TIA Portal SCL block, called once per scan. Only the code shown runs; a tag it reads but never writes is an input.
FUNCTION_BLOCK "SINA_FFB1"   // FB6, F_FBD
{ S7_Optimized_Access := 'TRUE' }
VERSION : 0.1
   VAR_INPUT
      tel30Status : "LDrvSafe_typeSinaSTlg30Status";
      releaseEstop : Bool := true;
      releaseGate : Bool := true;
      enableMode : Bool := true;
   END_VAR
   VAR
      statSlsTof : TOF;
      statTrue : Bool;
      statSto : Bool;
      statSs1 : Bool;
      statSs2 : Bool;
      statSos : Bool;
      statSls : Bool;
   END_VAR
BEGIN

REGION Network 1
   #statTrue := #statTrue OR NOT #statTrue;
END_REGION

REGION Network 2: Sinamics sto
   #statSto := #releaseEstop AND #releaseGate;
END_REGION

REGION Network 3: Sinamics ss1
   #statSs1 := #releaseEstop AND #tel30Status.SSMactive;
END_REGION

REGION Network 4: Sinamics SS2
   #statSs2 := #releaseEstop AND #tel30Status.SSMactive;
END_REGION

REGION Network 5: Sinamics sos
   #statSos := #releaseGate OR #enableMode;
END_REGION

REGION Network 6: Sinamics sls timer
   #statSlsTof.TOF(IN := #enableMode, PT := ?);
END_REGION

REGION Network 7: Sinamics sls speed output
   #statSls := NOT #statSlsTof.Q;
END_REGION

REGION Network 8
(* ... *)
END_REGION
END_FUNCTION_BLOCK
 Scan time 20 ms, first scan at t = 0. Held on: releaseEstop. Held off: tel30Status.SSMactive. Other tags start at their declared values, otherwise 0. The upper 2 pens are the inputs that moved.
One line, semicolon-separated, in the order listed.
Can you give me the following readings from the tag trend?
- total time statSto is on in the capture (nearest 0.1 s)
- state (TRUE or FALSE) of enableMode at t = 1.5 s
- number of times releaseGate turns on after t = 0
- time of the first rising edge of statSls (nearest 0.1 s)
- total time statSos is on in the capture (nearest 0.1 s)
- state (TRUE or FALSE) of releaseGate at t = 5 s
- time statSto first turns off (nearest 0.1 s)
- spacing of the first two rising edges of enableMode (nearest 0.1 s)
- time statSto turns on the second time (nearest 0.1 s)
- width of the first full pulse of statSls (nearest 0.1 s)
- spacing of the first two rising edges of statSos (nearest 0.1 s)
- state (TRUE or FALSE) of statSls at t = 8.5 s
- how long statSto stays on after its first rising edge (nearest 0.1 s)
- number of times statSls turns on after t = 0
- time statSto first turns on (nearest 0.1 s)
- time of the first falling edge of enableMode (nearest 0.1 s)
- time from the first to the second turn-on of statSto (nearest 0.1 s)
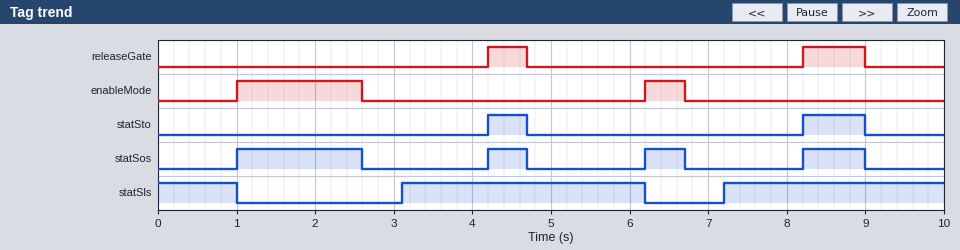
1.3 s; TRUE; 2; 3.1 s; 3.4 s; FALSE; 4.7 s; 5.2 s; 8.2 s; 3.1 s; 3.2 s; TRUE; 0.5 s; 2; 4.2 s; 2.6 s; 4.0 s
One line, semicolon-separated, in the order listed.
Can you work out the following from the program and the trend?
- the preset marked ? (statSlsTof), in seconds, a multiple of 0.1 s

0.5 s
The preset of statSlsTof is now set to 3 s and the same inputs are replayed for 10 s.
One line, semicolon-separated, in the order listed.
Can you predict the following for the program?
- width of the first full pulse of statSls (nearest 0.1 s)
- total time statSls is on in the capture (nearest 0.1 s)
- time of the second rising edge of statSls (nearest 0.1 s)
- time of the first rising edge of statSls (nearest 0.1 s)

0.6 s; 1.9 s; 9.7 s; 5.6 s
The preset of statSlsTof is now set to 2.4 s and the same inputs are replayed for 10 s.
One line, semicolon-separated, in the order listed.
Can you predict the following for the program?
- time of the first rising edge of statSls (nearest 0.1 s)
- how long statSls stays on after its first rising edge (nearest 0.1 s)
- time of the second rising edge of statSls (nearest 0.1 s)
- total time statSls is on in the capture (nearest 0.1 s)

5.0 s; 1.2 s; 9.1 s; 3.1 s
